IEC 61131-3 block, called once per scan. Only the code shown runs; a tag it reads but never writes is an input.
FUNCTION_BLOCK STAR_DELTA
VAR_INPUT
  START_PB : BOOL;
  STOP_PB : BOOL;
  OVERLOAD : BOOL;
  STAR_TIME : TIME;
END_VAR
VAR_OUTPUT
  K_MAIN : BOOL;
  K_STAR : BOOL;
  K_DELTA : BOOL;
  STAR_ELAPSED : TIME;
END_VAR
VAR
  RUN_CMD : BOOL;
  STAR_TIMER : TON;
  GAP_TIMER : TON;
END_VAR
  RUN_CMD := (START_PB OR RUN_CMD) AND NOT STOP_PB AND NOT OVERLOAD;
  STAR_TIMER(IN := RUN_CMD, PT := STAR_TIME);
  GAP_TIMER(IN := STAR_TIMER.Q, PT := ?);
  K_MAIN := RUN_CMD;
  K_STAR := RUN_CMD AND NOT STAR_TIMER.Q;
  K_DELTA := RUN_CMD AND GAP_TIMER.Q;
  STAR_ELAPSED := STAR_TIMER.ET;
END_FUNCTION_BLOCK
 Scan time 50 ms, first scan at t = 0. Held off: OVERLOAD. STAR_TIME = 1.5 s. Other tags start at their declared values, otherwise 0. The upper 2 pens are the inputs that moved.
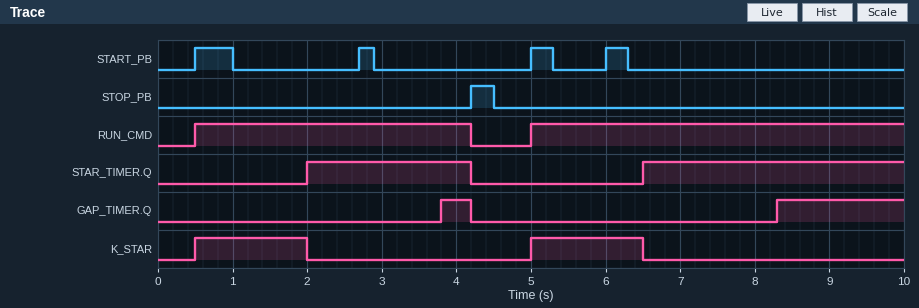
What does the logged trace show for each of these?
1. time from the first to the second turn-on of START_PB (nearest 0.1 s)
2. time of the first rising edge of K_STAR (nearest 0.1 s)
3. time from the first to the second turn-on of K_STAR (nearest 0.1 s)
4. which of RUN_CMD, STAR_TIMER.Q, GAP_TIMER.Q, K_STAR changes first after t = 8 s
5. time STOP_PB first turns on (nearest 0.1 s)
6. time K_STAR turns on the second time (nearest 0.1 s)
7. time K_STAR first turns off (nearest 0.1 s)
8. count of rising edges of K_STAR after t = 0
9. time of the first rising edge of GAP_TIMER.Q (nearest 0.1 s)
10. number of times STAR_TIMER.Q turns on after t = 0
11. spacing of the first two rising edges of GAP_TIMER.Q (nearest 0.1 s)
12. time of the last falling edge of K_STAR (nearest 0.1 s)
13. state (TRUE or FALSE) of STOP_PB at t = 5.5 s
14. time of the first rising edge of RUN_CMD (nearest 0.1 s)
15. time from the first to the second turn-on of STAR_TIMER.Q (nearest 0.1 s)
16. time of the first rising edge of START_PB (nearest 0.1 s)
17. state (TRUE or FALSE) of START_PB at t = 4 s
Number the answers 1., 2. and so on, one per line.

1. 2.2 s
2. 0.5 s
3. 4.5 s
4. GAP_TIMER.Q
5. 4.2 s
6. 5.0 s
7. 2.0 s
8. 2
9. 3.8 s
10. 2
11. 4.5 s
12. 6.5 s
13. FALSE
14. 0.5 s
15. 4.5 s
16. 0.5 s
17. FALSE
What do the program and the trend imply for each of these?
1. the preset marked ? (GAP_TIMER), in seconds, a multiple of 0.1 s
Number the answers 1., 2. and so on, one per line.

1. 1.8 s
